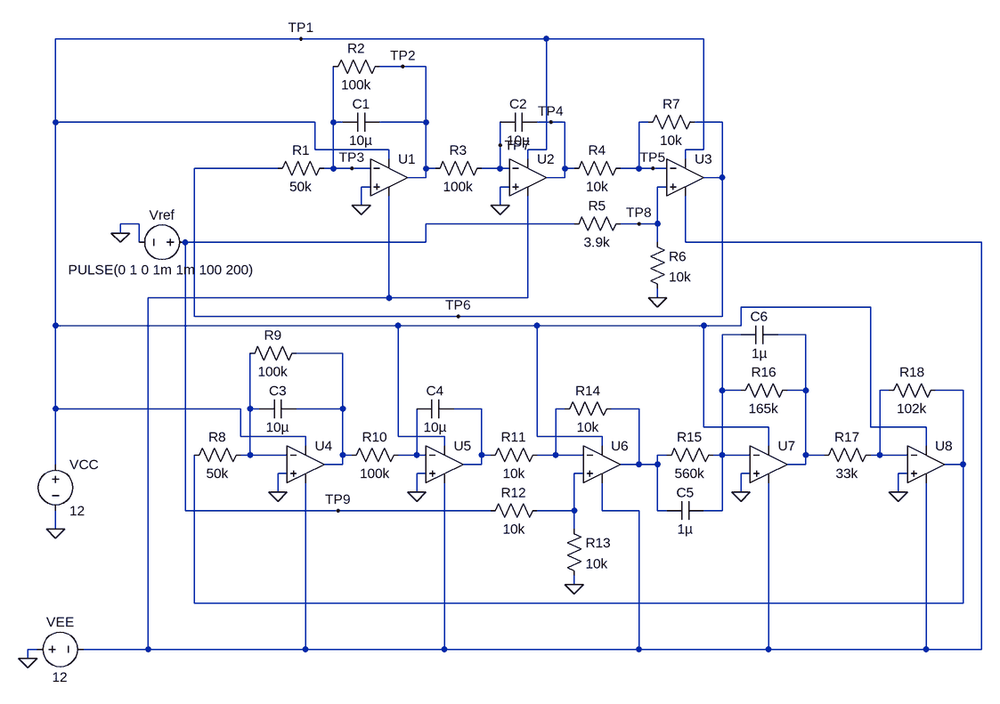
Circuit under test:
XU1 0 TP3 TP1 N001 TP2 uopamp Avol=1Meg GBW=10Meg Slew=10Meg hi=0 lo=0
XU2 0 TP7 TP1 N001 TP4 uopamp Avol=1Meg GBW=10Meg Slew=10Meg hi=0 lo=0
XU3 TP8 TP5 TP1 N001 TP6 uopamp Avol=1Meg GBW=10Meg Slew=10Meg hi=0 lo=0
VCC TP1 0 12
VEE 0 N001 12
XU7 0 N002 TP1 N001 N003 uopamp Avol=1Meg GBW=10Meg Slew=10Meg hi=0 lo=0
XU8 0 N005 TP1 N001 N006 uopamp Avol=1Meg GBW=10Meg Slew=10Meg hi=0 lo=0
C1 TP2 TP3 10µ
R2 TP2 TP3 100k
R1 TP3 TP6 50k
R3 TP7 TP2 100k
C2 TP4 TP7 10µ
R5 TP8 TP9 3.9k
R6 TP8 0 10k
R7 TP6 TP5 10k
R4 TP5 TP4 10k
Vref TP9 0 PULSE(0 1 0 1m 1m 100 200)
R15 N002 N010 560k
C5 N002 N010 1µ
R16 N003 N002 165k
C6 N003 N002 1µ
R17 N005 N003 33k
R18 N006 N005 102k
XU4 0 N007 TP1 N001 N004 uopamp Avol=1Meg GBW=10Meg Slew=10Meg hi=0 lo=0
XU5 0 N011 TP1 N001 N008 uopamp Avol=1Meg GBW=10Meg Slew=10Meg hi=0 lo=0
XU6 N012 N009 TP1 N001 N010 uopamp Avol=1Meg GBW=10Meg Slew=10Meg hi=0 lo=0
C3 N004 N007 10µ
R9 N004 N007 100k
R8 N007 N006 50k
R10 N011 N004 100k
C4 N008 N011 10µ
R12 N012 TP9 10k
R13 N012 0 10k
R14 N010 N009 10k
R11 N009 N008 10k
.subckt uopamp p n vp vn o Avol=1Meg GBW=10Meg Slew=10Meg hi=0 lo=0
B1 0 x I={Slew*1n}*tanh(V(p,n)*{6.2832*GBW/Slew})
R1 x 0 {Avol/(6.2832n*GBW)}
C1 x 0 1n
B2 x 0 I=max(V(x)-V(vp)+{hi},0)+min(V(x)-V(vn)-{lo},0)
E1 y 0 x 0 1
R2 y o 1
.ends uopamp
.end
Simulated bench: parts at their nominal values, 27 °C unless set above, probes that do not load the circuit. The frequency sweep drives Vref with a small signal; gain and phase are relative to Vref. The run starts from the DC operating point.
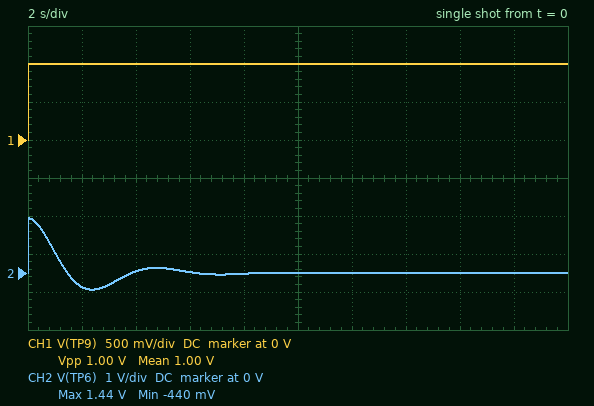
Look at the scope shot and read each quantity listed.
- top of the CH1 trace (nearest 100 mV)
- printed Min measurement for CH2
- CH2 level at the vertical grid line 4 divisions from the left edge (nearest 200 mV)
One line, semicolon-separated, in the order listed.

1.0 V; -440 mV; 0 V
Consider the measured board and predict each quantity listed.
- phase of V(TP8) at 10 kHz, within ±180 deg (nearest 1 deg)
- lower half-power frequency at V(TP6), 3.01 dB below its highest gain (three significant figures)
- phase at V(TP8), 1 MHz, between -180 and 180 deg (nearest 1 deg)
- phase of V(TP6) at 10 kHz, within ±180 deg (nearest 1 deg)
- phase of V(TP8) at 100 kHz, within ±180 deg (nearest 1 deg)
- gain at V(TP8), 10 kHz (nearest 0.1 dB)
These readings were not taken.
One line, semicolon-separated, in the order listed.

0 deg; 179 mHz; 0 deg; 0 deg; 0 deg; -2.9 dB
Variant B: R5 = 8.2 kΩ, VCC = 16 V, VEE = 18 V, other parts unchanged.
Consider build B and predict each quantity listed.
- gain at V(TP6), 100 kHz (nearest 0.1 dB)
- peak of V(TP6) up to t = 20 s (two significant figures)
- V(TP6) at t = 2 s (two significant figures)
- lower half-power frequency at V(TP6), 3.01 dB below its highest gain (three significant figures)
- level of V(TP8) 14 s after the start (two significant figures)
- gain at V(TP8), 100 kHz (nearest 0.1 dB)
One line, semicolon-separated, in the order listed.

0.8 dB; 1.1 V; -280 mV; 179 mHz; 550 mV; -5.2 dB
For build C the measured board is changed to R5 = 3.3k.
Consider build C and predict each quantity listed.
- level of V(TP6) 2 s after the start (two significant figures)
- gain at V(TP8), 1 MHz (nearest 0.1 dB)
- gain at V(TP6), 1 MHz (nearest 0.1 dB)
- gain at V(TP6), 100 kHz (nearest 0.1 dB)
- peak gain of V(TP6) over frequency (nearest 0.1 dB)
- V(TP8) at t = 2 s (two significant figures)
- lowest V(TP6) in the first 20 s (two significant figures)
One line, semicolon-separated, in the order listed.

-390 mV; -2.5 dB; 3.4 dB; 3.5 dB; 8.6 dB; 750 mV; -460 mV
